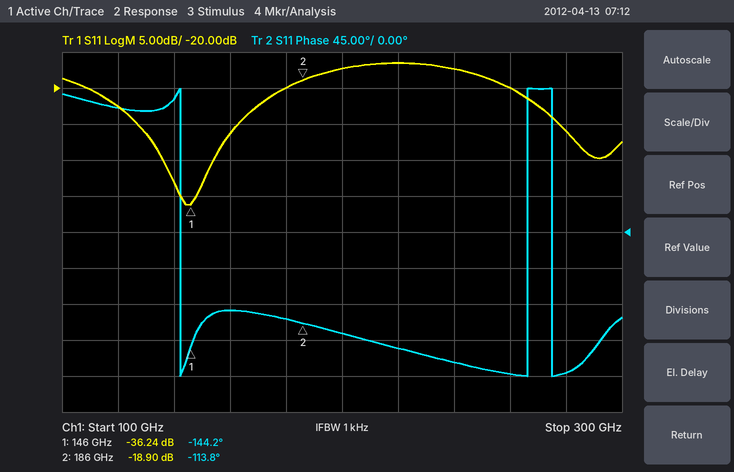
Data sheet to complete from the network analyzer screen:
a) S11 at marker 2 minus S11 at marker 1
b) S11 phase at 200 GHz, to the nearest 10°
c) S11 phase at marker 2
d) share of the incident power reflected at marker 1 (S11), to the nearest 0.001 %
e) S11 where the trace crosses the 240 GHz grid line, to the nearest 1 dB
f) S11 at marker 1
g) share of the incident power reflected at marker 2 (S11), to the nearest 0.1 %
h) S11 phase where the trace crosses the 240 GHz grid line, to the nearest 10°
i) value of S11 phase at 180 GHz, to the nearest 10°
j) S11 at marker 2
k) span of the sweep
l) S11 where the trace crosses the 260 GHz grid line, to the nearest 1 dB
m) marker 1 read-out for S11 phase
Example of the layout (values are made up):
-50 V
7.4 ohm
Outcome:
17.34 dB
-130°
-113.8°
0.024 %
-17 dB
-36.24 dB
1.3 %
-160°
-110°
-18.90 dB
200 GHz
-20 dB
-144.2°
